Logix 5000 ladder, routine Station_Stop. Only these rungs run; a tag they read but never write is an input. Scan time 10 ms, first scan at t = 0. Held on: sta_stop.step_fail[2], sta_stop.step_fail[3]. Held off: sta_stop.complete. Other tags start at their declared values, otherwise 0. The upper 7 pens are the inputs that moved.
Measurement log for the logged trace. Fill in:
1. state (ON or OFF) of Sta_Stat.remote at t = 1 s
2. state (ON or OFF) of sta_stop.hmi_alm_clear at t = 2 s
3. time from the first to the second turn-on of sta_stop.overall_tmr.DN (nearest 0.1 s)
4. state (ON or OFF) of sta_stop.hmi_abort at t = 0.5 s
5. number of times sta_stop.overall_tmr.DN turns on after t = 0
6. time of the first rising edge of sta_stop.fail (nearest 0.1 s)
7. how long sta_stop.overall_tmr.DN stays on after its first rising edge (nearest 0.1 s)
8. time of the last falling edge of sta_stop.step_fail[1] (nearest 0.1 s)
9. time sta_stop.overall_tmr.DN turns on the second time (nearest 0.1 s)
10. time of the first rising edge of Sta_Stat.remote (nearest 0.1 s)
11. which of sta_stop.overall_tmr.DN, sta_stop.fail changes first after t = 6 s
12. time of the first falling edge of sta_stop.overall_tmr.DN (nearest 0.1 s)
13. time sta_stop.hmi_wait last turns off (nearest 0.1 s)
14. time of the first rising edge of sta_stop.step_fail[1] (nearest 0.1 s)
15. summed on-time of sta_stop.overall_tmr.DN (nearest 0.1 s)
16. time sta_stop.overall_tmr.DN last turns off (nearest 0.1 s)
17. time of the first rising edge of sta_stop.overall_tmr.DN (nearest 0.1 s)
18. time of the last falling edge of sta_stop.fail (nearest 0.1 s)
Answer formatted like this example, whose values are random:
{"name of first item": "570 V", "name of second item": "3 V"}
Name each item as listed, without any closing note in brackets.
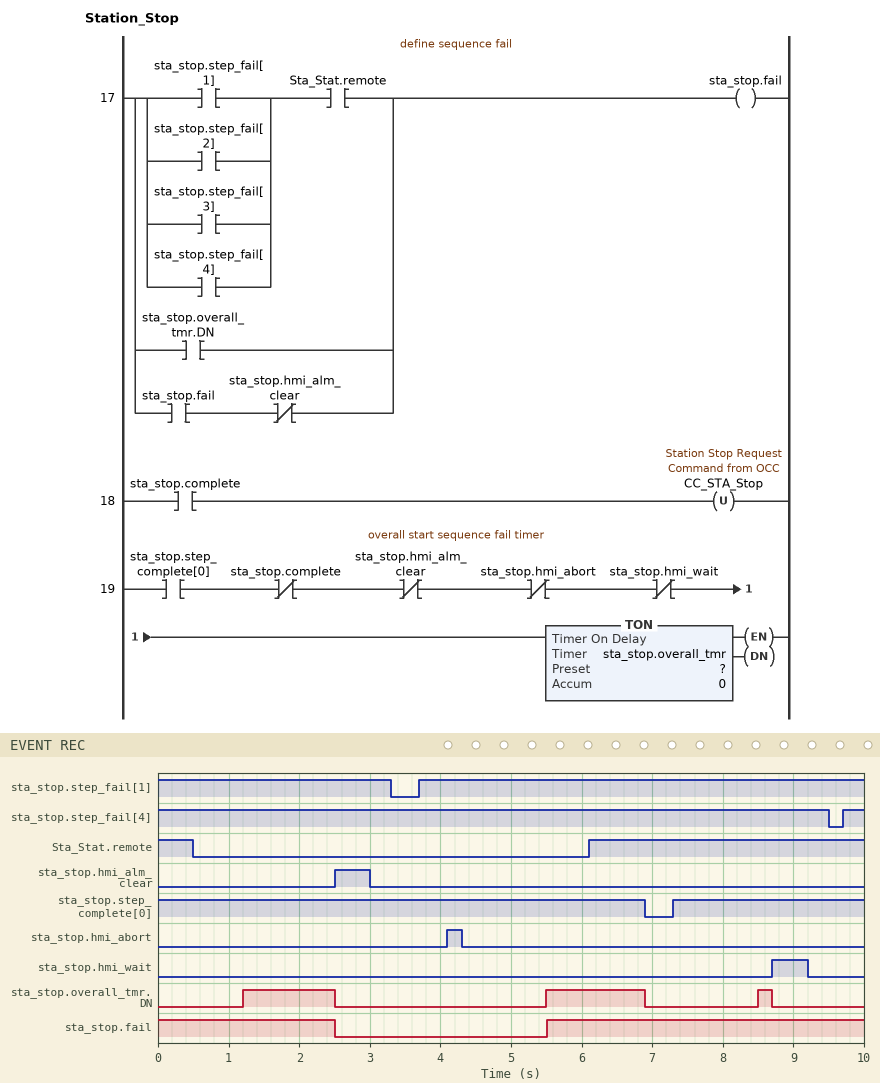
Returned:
{"state (ON or OFF) of Sta_Stat.remote at t = 1 s": "OFF", "state (ON or OFF) of sta_stop.hmi_alm_clear at t = 2 s": "OFF", "time from the first to the second turn-on of sta_stop.overall_tmr.DN": "4.3 s", "state (ON or OFF) of sta_stop.hmi_abort at t = 0.5 s": "OFF", "number of times sta_stop.overall_tmr.DN turns on after t = 0": "3", "time of the first rising edge of sta_stop.fail": "5.5 s", "how long sta_stop.overall_tmr.DN stays on after its first rising edge": "1.3 s", "time of the last falling edge of sta_stop.step_fail[1]": "3.3 s", "time sta_stop.overall_tmr.DN turns on the second time": "5.5 s", "time of the first rising edge of Sta_Stat.remote": "6.1 s", "which of sta_stop.overall_tmr.DN, sta_stop.fail changes first after t = 6 s": "sta_stop.overall_tmr.DN", "time of the first falling edge of sta_stop.overall_tmr.DN": "2.5 s", "time sta_stop.hmi_wait last turns off": "9.2 s", "time of the first rising edge of sta_stop.step_fail[1]": "3.7 s", "summed on-time of sta_stop.overall_tmr.DN": "2.9 s", "time sta_stop.overall_tmr.DN last turns off": "8.7 s", "time of the first rising edge of sta_stop.overall_tmr.DN": "1.2 s", "time of the last falling edge of sta_stop.fail": "2.5 s"}
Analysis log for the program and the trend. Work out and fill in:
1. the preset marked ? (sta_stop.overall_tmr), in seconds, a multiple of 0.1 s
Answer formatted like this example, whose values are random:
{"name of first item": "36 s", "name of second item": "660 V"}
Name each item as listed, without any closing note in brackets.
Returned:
{"the preset marked ? (sta_stop.overall_tmr), in seconds, a multiple of 0.1 s": "1.2 s"}
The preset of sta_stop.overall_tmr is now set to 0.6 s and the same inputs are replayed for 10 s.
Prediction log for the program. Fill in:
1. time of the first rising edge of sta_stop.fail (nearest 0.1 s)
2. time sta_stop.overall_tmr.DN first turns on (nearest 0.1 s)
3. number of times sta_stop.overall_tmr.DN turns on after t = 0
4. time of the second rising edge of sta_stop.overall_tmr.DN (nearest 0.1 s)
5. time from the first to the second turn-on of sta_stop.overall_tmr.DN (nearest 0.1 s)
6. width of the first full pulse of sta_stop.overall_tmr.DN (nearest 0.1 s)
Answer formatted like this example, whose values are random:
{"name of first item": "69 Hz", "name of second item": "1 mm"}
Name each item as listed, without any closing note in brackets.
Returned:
{"time of the first rising edge of sta_stop.fail": "3.6 s", "time sta_stop.overall_tmr.DN first turns on": "0.6 s", "number of times sta_stop.overall_tmr.DN turns on after t = 0": "5", "time of the second rising edge of sta_stop.overall_tmr.DN": "3.6 s", "time from the first to the second turn-on of sta_stop.overall_tmr.DN": "3.0 s", "width of the first full pulse of sta_stop.overall_tmr.DN": "1.9 s"}
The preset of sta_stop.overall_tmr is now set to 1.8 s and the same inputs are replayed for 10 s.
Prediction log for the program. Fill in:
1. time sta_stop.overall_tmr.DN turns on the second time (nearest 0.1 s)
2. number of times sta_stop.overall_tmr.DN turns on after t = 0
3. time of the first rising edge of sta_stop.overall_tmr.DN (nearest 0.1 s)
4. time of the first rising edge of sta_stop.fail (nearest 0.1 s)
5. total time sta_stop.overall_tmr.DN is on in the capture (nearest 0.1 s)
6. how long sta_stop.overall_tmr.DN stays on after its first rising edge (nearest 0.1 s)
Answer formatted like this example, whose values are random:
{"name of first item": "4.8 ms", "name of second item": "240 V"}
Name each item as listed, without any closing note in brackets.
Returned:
{"time sta_stop.overall_tmr.DN turns on the second time": "6.1 s", "number of times sta_stop.overall_tmr.DN turns on after t = 0": "2", "time of the first rising edge of sta_stop.overall_tmr.DN": "1.8 s", "time of the first rising edge of sta_stop.fail": "6.1 s", "total time sta_stop.overall_tmr.DN is on in the capture": "1.5 s", "how long sta_stop.overall_tmr.DN stays on after its first rising edge": "0.7 s"}
